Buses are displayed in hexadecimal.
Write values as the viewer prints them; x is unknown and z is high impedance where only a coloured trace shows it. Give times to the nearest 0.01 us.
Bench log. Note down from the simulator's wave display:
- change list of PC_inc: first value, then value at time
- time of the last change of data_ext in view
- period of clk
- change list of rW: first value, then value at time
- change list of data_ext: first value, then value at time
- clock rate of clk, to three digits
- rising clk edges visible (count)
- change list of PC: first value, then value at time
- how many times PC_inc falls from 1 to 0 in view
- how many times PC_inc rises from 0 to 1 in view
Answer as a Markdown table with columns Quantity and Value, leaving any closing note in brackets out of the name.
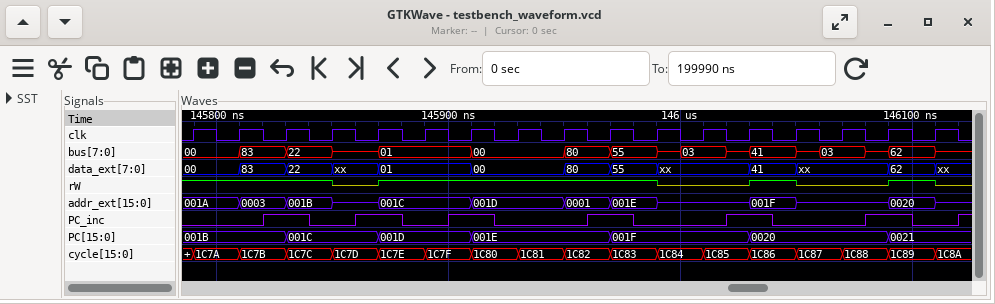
| Quantity | Value |
|---|---|
| change list of PC_inc: first value, then value at time | 0, 1 at 145.82 us, 0 at 145.84 us, 1 at 145.86 us, 0 at 145.88 us, 1 at 145.9 us, 0 at 145.92 us, 1 at 145.96 us, 0 at 145.98 us, 1 at 146.02 us, 0 at 146.04 us, 1 at 146.08 us, 0 at 146.1 us, 1 at 146.12 us |
| time of the last change of data_ext in view | 146.11 us |
| period of clk | 0.02 us |
| change list of rW: first value, then value at time | 1, z at 145.85 us, 1 at 145.87 us, z at 145.99 us, 1 at 146.03 us, z at 146.05 us, 1 at 146.09 us, z at 146.11 us |
| change list of data_ext: first value, then value at time | 00, 83 at 145.81 us, 22 at 145.83 us, xx at 145.85 us, 01 at 145.87 us, 00 at 145.91 us, 80 at 145.95 us, 55 at 145.97 us, xx at 145.99 us, 41 at 146.03 us, xx at 146.05 us, 62 at 146.09 us, xx at 146.11 us |
| clock rate of clk, to three digits | 50.0 MHz |
| rising clk edges visible | 17 |
| change list of PC: first value, then value at time | 001B, 001C at 145.83 us, 001D at 145.87 us, 001E at 145.91 us, 001F at 145.97 us, 0020 at 146.03 us, 0021 at 146.09 us |
| how many times PC_inc falls from 1 to 0 in view | 6 |
| how many times PC_inc rises from 0 to 1 in view | 7 |
